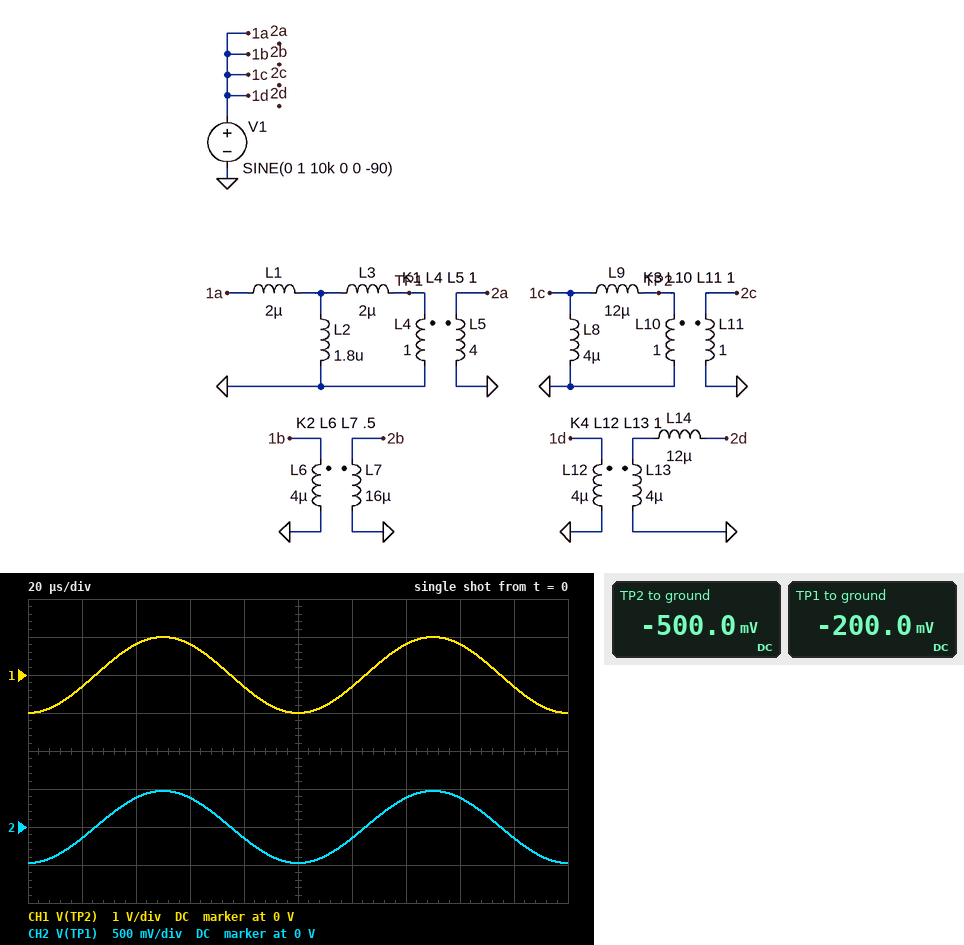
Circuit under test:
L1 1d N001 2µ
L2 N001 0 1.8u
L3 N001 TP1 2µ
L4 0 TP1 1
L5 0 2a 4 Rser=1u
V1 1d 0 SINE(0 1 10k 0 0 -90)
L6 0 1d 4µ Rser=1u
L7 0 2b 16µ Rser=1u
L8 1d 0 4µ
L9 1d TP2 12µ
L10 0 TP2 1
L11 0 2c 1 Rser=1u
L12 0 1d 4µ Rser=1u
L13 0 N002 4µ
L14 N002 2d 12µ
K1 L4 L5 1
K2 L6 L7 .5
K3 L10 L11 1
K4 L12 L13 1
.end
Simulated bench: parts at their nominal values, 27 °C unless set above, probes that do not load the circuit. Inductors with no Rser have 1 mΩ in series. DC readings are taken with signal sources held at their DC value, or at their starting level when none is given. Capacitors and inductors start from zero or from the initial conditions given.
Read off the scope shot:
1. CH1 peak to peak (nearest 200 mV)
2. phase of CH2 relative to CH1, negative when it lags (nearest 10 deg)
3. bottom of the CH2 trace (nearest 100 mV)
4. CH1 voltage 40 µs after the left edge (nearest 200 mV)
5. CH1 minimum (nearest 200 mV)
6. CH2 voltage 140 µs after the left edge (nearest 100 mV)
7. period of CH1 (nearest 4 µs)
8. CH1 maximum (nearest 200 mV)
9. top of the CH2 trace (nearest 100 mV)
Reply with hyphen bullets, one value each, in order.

- 2.0 V
- 0 deg
- -500 mV
- 800 mV
- -1.0 V
- 400 mV
- 100 µs
- 1.0 V
- 500 mV
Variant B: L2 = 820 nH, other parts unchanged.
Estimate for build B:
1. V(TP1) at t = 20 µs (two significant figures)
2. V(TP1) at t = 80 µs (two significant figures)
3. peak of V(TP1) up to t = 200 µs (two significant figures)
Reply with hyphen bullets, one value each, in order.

- -92 mV
- -88 mV
- 290 mV
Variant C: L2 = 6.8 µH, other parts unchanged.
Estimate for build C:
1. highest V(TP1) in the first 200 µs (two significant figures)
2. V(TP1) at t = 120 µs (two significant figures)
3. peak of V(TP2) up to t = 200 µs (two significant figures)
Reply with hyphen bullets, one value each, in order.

- 770 mV
- -240 mV
- 1.0 V
